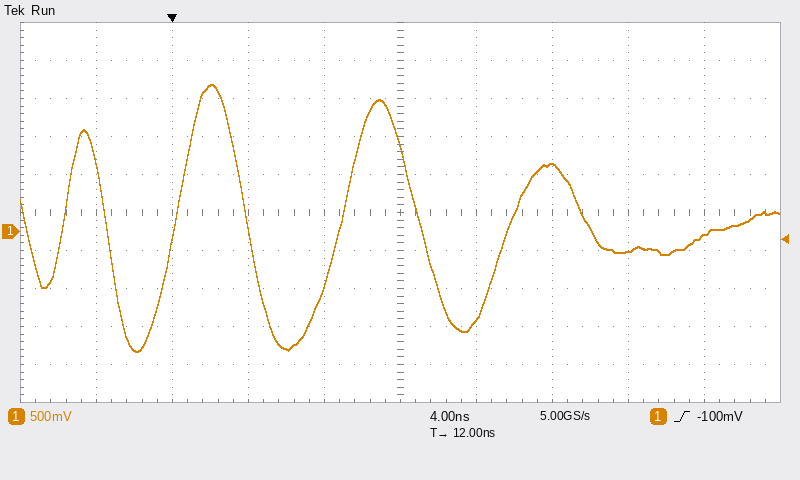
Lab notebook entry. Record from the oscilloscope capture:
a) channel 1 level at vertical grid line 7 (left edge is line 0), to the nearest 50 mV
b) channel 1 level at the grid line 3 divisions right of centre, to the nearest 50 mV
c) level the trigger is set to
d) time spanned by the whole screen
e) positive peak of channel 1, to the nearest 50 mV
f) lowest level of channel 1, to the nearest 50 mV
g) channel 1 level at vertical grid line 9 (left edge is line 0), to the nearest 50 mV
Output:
900 mV
-250 mV
-100 mV
40 ns
1.95 V
-1.60 V
-50 mV
